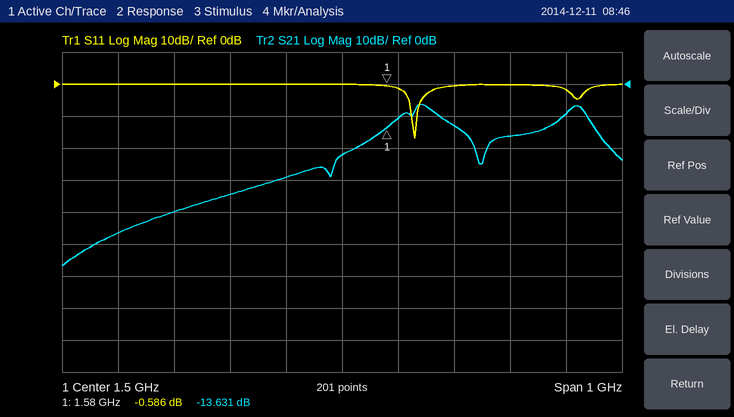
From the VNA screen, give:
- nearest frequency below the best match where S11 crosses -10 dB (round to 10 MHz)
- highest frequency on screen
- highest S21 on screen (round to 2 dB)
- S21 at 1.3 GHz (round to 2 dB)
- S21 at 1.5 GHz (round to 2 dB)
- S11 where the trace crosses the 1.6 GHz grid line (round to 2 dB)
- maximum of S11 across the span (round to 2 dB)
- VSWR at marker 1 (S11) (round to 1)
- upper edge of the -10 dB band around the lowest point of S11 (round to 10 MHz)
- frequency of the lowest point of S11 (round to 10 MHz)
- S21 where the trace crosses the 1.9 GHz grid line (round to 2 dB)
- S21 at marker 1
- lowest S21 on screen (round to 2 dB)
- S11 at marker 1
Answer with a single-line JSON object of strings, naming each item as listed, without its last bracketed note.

{"nearest frequency below the best match where S11 crosses -10 dB": "1.62 GHz", "highest frequency on screen": "2 GHz", "highest S21 on screen": "-6 dB", "S21 at 1.3 GHz": "-34 dB", "S21 at 1.5 GHz": "-22 dB", "S11 where the trace crosses the 1.6 GHz grid line": "-2 dB", "maximum of S11 across the span": "0 dB", "VSWR at marker 1 (S11)": "30", "upper edge of the -10 dB band around the lowest point of S11": "1.63 GHz", "frequency of the lowest point of S11": "1.63 GHz", "S21 where the trace crosses the 1.9 GHz grid line": "-10 dB", "S21 at marker 1": "-13.631 dB", "lowest S21 on screen": "-56 dB", "S11 at marker 1": "-0.586 dB"}
